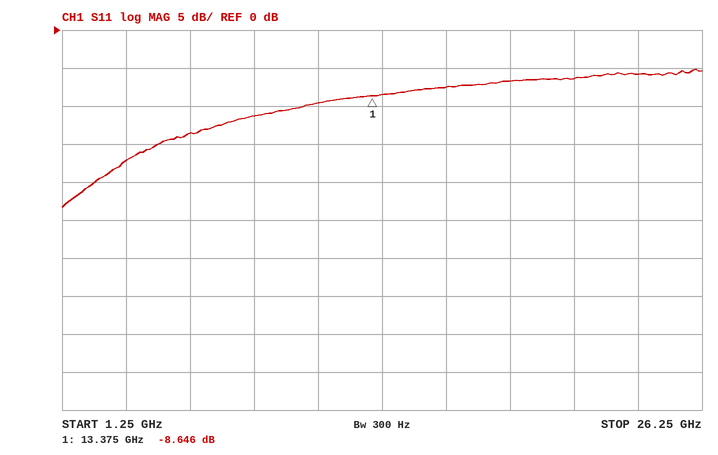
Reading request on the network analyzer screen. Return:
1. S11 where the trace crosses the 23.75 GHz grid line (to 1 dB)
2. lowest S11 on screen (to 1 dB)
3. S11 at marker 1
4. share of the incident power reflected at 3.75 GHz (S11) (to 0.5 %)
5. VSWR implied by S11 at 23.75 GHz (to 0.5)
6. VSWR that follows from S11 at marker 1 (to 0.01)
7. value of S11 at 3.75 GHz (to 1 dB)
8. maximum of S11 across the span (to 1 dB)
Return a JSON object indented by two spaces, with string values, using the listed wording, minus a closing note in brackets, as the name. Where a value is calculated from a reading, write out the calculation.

{
  "S11 where the trace crosses the 23.75 GHz grid line": "-6 dB",
  "lowest S11 on screen": "-23 dB",
  "S11 at marker 1": "-8.646 dB",
  "share of the incident power reflected at 3.75 GHz (S11)": "10^(-17/10) ≈ 2.0 %",
  "VSWR implied by S11 at 23.75 GHz": "|Γ| = 10^(-6/20) = 0.5012; VSWR = (1 + 0.5012)/(1 − 0.5012) ≈ 3.0",
  "VSWR that follows from S11 at marker 1": "(1 + 0.3696)/(1 − 0.3696) ≈ 2.17",
  "value of S11 at 3.75 GHz": "-17 dB",
  "maximum of S11 across the span": "-5 dB"
}
